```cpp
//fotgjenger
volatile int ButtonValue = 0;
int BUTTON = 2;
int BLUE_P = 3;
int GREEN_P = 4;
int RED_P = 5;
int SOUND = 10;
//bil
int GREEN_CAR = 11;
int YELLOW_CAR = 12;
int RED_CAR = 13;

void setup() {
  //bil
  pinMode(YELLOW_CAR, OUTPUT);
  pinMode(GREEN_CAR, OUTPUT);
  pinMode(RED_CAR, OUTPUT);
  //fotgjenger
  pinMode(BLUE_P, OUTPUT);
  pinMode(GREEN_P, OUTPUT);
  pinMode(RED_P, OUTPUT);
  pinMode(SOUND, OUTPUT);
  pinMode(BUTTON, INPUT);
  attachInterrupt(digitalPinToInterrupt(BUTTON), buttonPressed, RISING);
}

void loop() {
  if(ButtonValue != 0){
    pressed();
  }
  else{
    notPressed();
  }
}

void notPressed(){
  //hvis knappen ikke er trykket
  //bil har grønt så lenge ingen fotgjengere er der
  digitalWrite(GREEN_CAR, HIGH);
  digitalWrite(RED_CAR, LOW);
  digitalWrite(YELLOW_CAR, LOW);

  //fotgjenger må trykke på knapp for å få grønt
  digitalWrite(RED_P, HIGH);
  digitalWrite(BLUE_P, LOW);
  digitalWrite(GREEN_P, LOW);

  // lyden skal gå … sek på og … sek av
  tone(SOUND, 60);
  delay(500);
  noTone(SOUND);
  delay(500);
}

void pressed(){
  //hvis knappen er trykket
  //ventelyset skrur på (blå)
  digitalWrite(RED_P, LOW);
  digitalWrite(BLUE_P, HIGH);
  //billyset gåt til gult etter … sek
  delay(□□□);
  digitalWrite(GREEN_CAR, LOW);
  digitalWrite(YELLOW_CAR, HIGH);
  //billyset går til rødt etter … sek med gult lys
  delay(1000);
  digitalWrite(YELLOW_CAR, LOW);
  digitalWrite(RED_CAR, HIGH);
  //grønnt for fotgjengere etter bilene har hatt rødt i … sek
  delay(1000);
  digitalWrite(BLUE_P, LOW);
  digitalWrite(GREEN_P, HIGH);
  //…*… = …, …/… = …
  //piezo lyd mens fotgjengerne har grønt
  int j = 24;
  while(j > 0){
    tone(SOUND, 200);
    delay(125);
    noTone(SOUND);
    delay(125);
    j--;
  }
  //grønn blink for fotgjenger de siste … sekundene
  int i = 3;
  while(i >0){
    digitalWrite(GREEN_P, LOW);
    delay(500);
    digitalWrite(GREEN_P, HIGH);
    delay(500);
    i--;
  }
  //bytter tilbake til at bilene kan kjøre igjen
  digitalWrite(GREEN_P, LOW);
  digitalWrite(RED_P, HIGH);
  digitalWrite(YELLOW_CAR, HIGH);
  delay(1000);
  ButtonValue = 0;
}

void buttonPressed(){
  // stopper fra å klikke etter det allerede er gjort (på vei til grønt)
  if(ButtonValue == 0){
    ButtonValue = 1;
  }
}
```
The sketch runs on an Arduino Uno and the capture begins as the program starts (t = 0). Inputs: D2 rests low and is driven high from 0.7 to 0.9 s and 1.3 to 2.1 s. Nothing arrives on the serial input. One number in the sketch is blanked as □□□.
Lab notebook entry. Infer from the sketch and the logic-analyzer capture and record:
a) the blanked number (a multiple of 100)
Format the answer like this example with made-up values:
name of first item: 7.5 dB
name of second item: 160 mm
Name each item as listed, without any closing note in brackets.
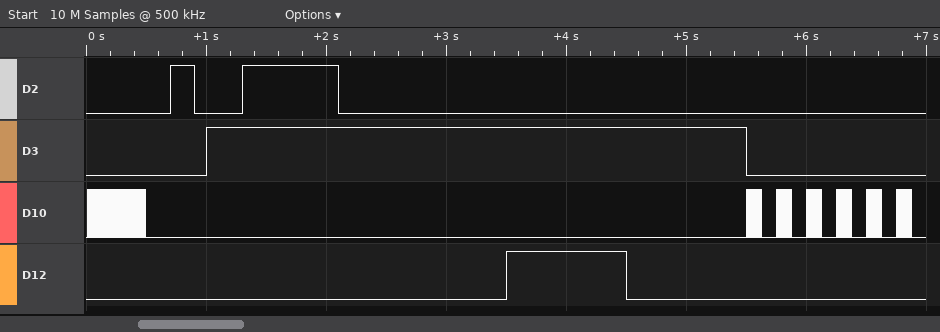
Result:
the blanked number: 2500
